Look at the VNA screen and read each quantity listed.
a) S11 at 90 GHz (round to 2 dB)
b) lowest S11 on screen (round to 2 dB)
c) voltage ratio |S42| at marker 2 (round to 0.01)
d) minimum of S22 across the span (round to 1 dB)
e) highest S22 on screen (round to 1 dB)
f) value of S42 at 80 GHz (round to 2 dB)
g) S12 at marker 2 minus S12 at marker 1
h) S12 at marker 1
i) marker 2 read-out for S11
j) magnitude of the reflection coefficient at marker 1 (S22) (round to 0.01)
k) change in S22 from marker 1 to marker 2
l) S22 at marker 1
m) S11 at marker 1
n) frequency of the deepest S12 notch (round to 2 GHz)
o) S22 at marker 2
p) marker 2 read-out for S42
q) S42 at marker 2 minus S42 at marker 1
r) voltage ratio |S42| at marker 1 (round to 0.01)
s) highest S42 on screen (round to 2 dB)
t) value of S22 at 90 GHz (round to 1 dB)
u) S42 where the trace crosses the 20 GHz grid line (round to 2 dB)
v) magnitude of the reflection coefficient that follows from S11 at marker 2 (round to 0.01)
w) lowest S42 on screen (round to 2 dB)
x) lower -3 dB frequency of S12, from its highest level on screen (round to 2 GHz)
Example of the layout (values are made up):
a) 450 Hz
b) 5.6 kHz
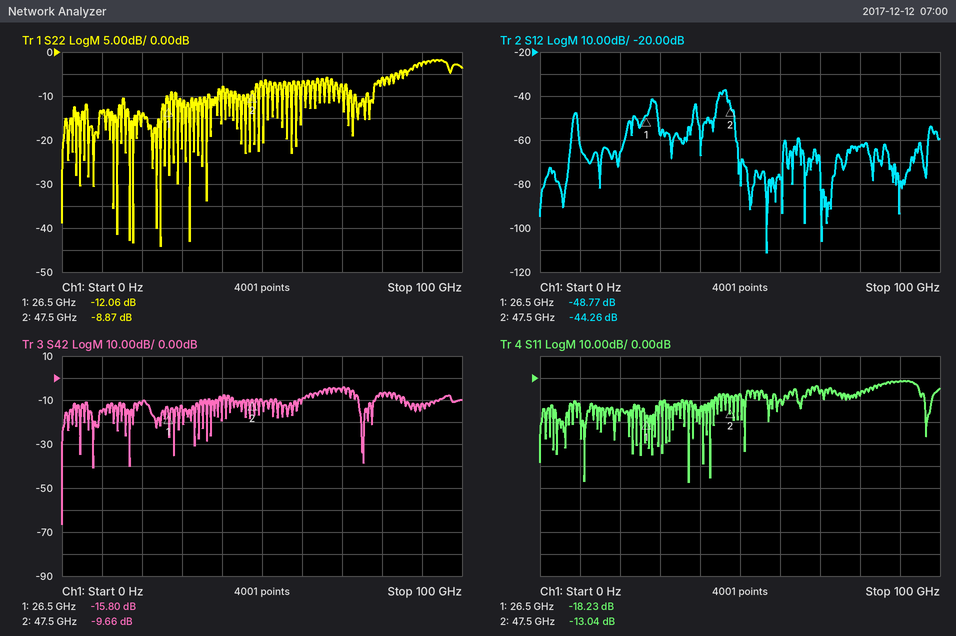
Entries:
a) -2 dB
b) -48 dB
c) 0.33
d) -44 dB
e) -2 dB
f) -8 dB
g) 4.51 dB
h) -48.77 dB
i) -13.04 dB
j) 0.25
k) 3.19 dB
l) -12.06 dB
m) -18.23 dB
n) 56 GHz
o) -8.87 dB
p) -9.66 dB
q) 6.14 dB
r) 0.16
s) -4 dB
t) -3 dB
u) -12 dB
v) 0.22
w) -66 dB
x) 44 GHz
